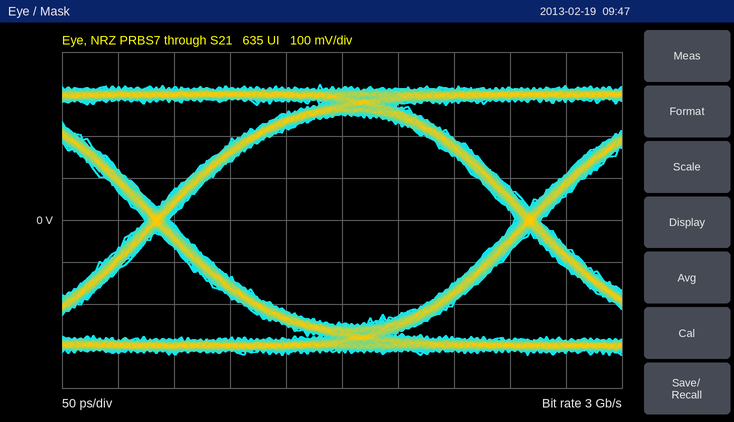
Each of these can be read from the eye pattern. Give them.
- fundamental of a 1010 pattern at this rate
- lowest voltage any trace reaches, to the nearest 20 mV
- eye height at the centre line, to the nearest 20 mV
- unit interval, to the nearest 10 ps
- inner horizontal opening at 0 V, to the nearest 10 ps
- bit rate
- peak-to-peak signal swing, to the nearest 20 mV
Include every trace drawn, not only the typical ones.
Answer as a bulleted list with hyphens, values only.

- 1.5 GHz
- -320 mV
- 500 mV
- 330 ps
- 310 ps
- 3 Gb/s
- 640 mV
